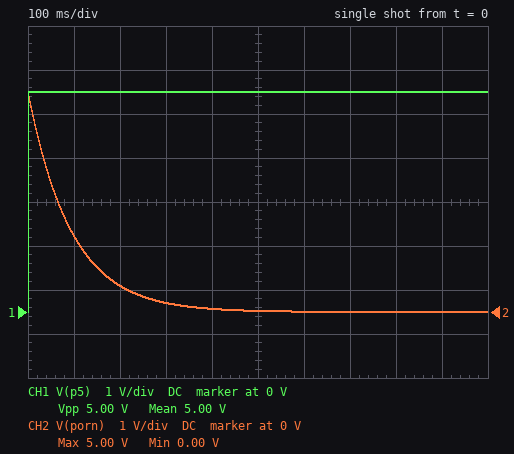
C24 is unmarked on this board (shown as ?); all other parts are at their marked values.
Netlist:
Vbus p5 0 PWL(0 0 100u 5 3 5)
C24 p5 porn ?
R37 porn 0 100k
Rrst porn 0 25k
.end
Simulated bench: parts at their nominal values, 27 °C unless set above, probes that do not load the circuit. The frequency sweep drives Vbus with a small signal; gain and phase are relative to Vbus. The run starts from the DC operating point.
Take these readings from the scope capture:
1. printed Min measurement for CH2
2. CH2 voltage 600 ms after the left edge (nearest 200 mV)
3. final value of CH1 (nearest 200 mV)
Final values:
0.00 V
0 V
5.0 V
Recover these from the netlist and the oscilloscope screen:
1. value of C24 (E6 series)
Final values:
4.7 µF
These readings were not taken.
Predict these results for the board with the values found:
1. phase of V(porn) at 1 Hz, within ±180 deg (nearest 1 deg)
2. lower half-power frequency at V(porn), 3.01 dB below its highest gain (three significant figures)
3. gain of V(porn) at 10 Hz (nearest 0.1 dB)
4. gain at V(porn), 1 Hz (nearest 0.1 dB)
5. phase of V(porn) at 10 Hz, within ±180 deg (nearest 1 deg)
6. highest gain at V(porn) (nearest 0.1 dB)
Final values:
59 deg
1.69 Hz
-0.1 dB
-5.9 dB
10 deg
0 dB
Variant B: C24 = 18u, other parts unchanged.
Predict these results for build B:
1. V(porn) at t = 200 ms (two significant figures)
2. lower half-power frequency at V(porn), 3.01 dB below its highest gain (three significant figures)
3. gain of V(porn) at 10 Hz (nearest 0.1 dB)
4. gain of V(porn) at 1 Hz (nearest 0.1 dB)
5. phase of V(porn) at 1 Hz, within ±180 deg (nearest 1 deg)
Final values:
2.9 V
442 mHz
0 dB
-0.8 dB
24 deg
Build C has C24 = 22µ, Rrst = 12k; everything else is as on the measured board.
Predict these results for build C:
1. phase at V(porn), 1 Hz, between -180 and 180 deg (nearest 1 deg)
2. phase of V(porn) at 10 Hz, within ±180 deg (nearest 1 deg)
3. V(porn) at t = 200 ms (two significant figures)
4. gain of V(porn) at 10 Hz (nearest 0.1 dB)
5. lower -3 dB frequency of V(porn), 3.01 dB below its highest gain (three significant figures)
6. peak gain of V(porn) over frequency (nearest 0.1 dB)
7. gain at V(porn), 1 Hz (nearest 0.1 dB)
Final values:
34 deg
4 deg
2.1 V
0 dB
675 mHz
0 dB
-1.6 dB
